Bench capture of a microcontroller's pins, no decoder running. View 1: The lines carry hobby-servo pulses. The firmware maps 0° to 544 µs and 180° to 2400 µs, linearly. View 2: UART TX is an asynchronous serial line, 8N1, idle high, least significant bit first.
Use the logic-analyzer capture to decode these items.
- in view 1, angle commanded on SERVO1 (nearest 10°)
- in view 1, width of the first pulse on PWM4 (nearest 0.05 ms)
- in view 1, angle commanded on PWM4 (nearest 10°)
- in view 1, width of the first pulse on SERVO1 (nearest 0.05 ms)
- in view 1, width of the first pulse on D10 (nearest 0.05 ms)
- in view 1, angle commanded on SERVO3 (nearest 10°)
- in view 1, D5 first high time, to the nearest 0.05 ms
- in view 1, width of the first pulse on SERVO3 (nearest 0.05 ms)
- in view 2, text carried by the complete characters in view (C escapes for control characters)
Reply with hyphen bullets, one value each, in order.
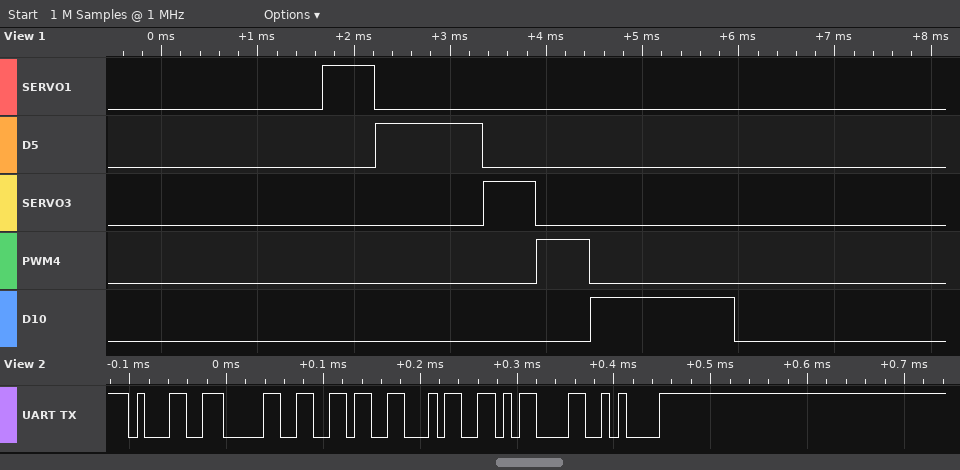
- 0°
- 0.55 ms
- 0°
- 0.55 ms
- 1.50 ms
- 0°
- 1.10 ms
- 0.55 ms
- "1064\r\n"
